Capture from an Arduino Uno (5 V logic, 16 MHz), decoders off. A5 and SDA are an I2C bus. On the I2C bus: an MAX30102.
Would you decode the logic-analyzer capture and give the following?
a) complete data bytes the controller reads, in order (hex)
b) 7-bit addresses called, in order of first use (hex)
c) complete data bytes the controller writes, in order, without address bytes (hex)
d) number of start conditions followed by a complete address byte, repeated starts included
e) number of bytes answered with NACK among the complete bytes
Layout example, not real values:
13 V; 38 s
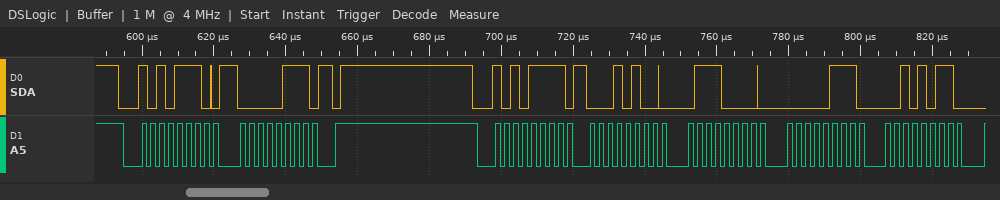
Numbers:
14 70 07 2B; 0x57; 07; 2; 0
